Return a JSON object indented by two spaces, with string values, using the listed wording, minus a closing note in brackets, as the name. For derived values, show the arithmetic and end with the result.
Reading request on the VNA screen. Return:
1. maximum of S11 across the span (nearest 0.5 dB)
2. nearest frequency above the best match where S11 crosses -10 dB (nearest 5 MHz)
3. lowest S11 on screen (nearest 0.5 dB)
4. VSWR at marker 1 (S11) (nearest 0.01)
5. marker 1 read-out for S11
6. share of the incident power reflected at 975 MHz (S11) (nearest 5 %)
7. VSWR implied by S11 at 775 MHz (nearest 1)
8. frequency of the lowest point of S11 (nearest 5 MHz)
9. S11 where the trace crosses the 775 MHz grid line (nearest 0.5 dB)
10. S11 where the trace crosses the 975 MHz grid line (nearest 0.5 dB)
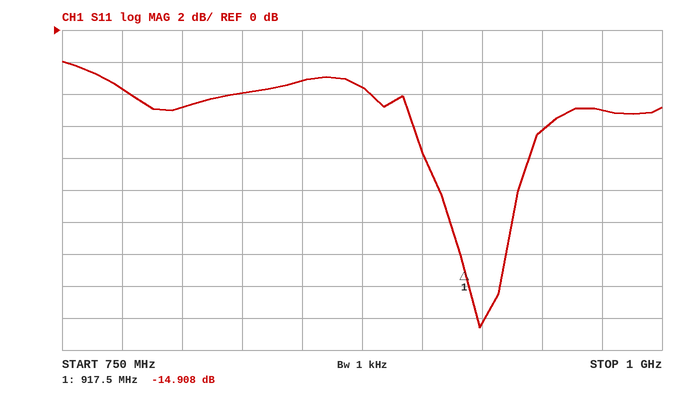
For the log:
{
  "maximum of S11 across the span": "-2.0 dB",
  "nearest frequency above the best match where S11 crosses -10 dB": "940 MHz",
  "lowest S11 on screen": "-18.5 dB",
  "VSWR at marker 1 (S11)": "(1 + 0.1797)/(1 − 0.1797) ≈ 1.44",
  "marker 1 read-out for S11": "-14.908 dB",
  "share of the incident power reflected at 975 MHz (S11)": "10^(-5/10) ≈ 31.6 %, so 30 % to the nearest 5 %",
  "VSWR implied by S11 at 775 MHz": "|Γ| = 10^(-3.5/20) = 0.6683; VSWR = (1 + 0.6683)/(1 − 0.6683) ≈ 5",
  "frequency of the lowest point of S11": "925 MHz",
  "S11 where the trace crosses the 775 MHz grid line": "-3.5 dB",
  "S11 where the trace crosses the 975 MHz grid line": "-5.0 dB"
}
